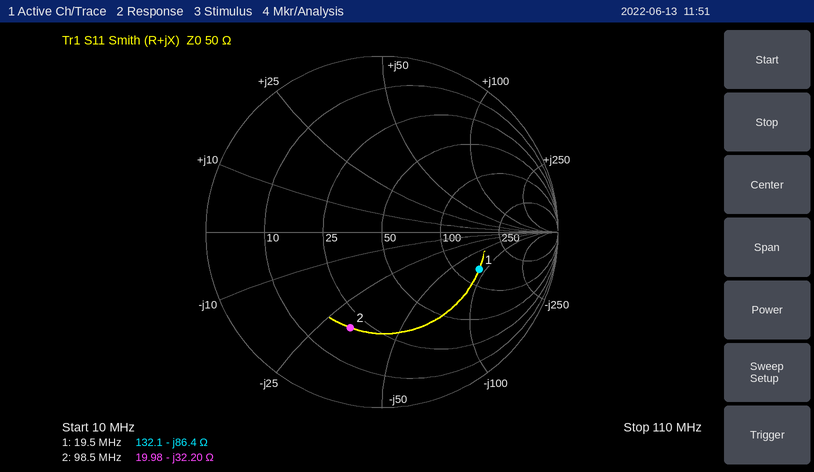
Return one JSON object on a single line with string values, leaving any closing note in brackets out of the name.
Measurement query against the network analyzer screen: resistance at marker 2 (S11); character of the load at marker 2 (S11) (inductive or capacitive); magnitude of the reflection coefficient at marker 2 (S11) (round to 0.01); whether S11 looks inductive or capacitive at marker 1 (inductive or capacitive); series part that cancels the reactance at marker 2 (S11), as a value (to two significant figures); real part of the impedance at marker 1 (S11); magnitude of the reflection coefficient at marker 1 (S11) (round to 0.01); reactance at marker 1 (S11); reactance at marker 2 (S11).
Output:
{"resistance at marker 2": "19.98 Ω", "character of the load at marker 2 (S11)": "capacitive", "magnitude of the reflection coefficient at marker 2 (S11)": "0.57", "whether S11 looks inductive or capacitive at marker 1": "capacitive", "series part that cancels the reactance at marker 2 (S11), as a value": "52 nH", "real part of the impedance at marker 1": "132.1 Ω", "magnitude of the reflection coefficient at marker 1 (S11)": "0.59", "reactance at marker 1": "-86.4 Ω", "reactance at marker 2": "-32.20 Ω"}
